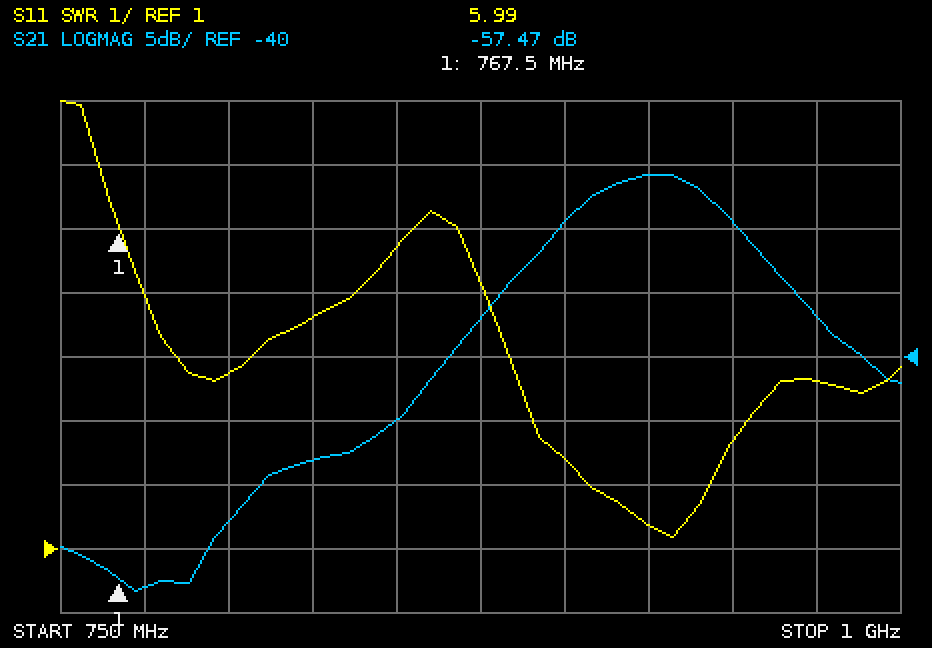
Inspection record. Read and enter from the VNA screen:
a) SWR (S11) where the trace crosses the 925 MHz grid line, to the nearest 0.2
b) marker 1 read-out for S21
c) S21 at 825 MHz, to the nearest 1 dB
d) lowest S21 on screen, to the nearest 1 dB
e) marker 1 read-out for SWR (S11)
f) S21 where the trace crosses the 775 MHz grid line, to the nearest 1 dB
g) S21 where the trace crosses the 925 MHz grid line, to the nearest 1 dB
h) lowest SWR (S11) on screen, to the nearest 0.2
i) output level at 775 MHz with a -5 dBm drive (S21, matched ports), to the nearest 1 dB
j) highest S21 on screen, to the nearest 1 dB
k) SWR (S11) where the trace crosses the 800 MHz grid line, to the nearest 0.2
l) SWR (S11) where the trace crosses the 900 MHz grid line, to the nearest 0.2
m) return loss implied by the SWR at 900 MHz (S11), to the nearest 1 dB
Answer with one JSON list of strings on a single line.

["1.4", "-57.47 dB", "-48 dB", "-58 dB", "5.99", "-58 dB", "-26 dB", "1.2", "-63 dBm", "-26 dB", "3.8", "2.4", "8 dB"]
